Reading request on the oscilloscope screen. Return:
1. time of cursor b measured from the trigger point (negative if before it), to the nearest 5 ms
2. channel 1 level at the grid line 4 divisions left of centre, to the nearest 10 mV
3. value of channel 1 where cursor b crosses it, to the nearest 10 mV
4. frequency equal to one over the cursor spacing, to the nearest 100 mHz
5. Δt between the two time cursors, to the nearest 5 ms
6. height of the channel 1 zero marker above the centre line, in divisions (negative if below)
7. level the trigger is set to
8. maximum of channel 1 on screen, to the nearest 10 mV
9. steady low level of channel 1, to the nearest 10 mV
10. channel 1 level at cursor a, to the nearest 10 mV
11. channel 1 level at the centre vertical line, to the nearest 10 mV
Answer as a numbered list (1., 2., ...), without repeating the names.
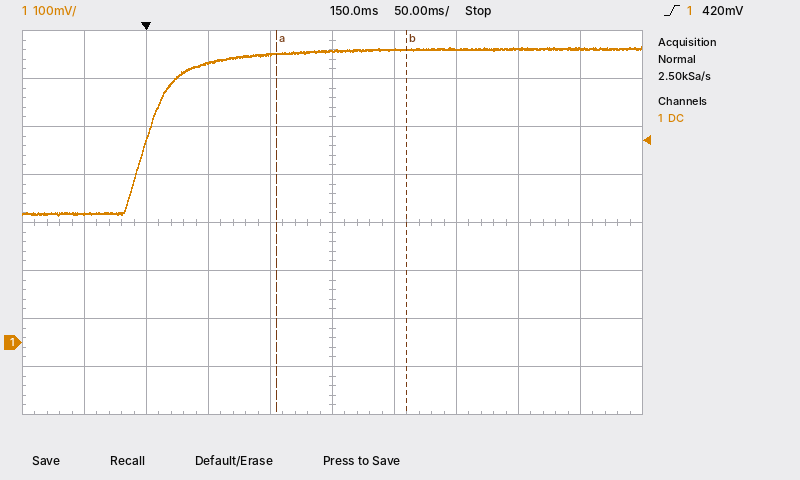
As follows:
1. +210 ms
2. 270 mV
3. 610 mV
4. 9.5 Hz
5. 105 ms
6. -2.5 div
7. 420 mV
8. 620 mV
9. 270 mV
10. 600 mV
11. 610 mV
